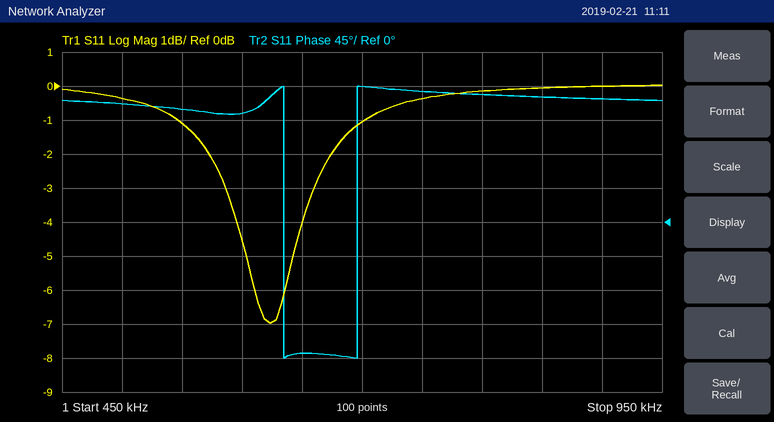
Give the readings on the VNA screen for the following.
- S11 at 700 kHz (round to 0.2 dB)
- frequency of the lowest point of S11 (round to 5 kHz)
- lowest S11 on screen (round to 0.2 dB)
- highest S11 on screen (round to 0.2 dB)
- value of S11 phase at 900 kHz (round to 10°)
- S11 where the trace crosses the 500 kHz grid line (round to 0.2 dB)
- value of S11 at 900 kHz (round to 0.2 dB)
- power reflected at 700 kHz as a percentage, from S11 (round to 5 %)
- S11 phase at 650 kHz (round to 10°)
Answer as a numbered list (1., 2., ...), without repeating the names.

1. -1.0 dB
2. 625 kHz
3. -7.0 dB
4. 0.0 dB
5. 160°
6. -0.4 dB
7. 0.0 dB
8. 80 %
9. -170°
